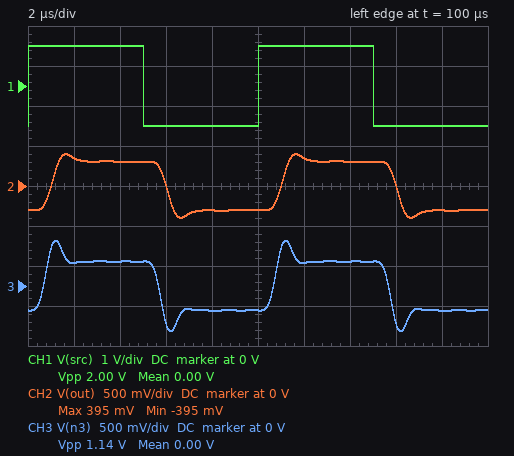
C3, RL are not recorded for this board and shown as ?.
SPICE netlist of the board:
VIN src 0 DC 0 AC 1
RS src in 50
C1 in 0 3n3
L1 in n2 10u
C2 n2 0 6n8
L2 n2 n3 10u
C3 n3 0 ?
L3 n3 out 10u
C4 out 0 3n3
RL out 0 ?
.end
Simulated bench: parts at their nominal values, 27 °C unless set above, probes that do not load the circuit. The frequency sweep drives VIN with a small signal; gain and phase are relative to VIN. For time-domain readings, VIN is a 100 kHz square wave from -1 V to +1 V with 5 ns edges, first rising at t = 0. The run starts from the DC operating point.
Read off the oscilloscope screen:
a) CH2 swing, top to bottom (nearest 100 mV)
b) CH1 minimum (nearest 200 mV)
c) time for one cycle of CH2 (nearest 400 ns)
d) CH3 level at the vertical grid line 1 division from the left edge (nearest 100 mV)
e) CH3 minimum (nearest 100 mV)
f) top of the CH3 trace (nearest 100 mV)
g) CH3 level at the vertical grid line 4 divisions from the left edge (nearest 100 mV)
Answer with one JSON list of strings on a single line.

["800 mV", "-1.0 V", "10.0 µs", "300 mV", "-600 mV", "600 mV", "-300 mV"]
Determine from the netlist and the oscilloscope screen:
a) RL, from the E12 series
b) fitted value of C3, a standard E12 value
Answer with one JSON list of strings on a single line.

["22 Ω", "18 nF"]
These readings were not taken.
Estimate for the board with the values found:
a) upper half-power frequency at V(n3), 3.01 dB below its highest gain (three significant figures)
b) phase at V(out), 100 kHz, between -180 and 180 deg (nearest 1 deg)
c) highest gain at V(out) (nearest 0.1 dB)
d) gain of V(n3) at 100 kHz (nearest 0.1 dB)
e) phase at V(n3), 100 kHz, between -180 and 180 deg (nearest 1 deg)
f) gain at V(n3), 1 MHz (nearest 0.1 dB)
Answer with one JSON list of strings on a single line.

["802 kHz", "-33 deg", "-9.8 dB", "-9.9 dB", "-17 deg", "-12.7 dB"]
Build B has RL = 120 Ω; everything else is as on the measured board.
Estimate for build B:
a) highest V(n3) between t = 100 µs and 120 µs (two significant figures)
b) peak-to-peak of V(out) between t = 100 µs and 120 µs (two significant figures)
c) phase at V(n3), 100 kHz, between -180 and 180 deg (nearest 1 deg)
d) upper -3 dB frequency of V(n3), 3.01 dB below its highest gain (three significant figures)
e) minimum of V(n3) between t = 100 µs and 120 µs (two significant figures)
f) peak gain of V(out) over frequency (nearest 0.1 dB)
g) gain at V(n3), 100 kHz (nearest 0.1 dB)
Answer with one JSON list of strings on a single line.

["700 mV", "1.4 V", "-40 deg", "209 kHz", "-700 mV", "-3.0 dB", "-4.1 dB"]
